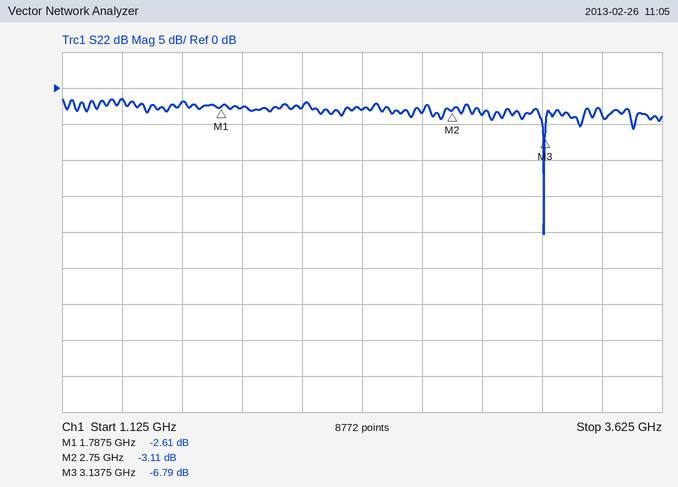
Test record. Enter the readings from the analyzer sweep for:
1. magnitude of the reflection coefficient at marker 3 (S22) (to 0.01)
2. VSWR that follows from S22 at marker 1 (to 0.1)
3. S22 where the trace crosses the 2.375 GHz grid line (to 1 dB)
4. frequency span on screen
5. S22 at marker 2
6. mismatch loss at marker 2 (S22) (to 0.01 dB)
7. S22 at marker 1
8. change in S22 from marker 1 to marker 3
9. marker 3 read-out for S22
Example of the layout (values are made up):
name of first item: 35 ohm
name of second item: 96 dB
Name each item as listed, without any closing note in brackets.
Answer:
magnitude of the reflection coefficient at marker 3 (S22): 0.46
VSWR that follows from S22 at marker 1: 6.7
S22 where the trace crosses the 2.375 GHz grid line: -3 dB
frequency span on screen: 2.5 GHz
S22 at marker 2: -3.11 dB
mismatch loss at marker 2 (S22): 2.91 dB
S22 at marker 1: -2.61 dB
change in S22 from marker 1 to marker 3: -4.18 dB
marker 3 read-out for S22: -6.79 dB
